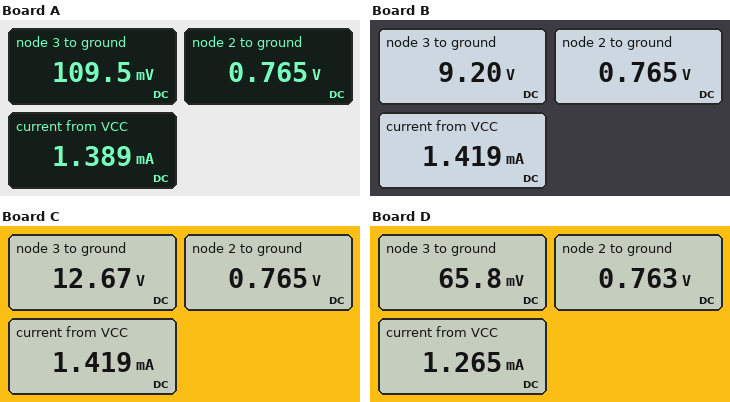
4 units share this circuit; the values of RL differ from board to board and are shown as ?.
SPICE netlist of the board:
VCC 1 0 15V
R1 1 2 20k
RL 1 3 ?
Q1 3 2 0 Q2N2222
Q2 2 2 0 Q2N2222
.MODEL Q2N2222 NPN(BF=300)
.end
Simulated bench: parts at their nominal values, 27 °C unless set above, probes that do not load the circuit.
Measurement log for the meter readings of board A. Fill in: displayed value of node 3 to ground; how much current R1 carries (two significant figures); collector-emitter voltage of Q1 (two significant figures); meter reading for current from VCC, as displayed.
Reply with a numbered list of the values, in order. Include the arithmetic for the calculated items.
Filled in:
1. 109.5 mV
2. (15 V - 765 mV) / 20 kΩ = 710 µA
3. 109.5 mV = 110 mV
4. 1.389 mA
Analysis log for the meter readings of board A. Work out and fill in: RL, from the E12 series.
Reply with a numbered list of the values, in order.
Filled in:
1. 22 kΩ
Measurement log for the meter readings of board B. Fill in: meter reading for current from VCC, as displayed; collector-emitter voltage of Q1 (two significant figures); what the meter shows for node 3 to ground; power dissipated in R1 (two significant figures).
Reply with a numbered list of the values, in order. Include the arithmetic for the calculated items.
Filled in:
1. 1.419 mA
2. 9.2 V = 9.2 V
3. 9.20 V
4. (15 V - 765 mV)^2 / 20 kΩ = 10 mW
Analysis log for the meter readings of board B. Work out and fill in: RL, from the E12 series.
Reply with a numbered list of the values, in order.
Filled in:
1. 8.2 kΩ
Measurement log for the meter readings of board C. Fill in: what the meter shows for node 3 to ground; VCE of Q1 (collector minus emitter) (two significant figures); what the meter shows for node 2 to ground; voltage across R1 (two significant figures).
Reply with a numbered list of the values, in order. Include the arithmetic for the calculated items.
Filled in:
1. 12.67 V
2. 12.67 V = 13 V
3. 0.765 V
4. 15 V - 765 mV = 14 V
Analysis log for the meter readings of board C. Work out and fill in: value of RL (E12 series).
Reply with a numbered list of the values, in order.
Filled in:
1. 3.3 kΩ
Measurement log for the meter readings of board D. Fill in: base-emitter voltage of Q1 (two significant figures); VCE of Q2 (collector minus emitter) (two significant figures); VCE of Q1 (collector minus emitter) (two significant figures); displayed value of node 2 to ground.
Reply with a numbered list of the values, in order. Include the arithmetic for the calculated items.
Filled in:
1. 763 mV = 760 mV
2. 763 mV = 760 mV
3. 65.8 mV = 66 mV
4. 0.763 V
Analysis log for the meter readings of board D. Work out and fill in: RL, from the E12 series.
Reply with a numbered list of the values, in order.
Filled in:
1. 27 kΩ
